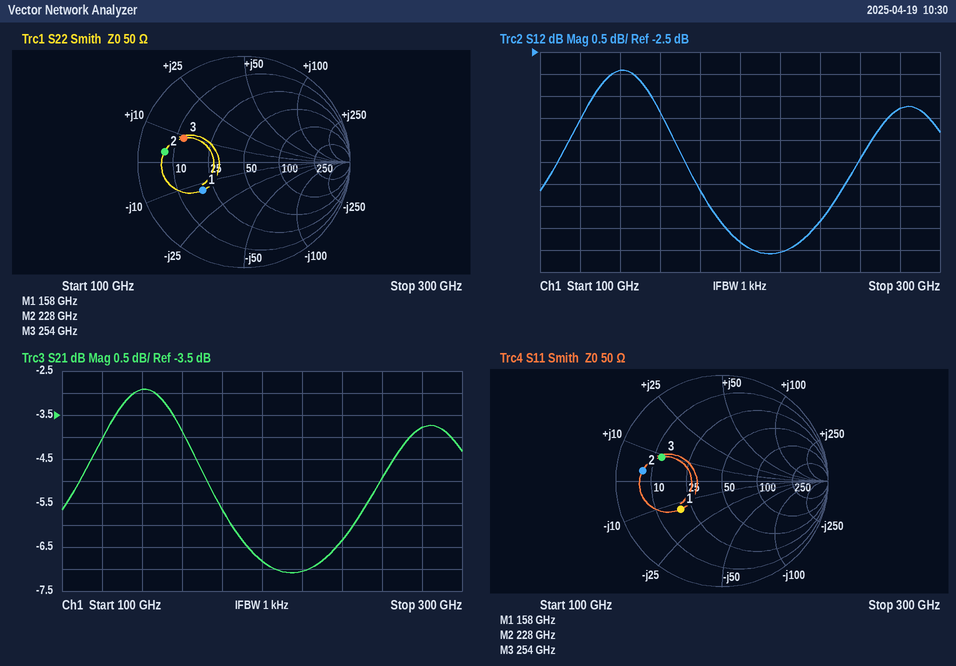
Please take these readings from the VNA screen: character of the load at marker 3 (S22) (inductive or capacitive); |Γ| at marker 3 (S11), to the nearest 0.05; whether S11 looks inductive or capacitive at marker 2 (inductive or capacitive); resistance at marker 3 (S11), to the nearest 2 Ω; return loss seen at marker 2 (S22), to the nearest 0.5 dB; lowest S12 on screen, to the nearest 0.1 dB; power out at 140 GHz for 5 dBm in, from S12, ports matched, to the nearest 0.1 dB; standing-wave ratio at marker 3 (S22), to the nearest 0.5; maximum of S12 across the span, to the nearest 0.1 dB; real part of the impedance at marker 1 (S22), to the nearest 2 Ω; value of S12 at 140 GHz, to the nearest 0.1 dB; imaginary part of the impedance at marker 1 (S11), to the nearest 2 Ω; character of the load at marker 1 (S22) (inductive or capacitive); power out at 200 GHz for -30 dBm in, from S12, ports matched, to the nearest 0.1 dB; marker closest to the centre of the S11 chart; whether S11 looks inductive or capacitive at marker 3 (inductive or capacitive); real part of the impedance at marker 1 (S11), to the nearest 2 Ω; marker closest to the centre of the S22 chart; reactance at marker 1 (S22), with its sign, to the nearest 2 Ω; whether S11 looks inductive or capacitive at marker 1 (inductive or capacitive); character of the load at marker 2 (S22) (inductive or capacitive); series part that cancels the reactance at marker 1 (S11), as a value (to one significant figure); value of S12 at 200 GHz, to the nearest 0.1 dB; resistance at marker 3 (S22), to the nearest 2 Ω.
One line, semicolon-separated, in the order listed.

inductive; 0.60; inductive; 12 Ω; 2.5 dB; -7.1 dB; 2.1 dBm; 4.0; -2.9 dB; 20 Ω; -2.9 dB; -14 Ω; capacitive; -36.8 dBm; marker 1; inductive; 20 Ω; marker 1; -14 Ω; capacitive; inductive; 10 pH; -6.8 dB; 12 Ω
